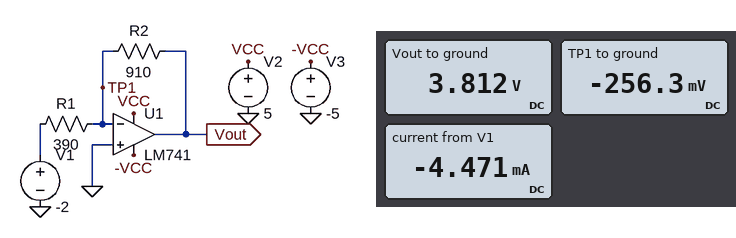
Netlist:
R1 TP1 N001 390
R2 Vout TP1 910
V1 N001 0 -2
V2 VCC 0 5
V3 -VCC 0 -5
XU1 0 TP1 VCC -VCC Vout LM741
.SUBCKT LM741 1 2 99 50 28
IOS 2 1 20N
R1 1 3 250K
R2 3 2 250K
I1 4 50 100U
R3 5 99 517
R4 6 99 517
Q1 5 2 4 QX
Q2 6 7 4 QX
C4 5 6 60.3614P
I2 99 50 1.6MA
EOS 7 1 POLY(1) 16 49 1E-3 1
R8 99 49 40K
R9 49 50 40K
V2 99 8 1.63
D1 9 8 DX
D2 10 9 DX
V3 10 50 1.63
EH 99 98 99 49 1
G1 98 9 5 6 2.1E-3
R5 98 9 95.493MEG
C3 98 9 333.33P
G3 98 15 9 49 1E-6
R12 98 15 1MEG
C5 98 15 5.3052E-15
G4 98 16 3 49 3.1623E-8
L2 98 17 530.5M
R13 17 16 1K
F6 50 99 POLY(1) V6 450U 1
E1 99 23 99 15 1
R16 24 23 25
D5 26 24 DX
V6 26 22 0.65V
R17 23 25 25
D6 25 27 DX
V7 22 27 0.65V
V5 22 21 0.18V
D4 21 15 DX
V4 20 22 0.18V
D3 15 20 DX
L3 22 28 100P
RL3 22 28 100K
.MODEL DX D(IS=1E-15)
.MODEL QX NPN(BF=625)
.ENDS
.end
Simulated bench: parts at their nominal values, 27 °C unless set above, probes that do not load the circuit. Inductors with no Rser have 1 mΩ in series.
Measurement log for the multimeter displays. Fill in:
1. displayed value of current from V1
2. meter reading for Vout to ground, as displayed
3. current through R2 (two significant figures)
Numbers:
-4.471 mA
3.812 V
4.5 mA
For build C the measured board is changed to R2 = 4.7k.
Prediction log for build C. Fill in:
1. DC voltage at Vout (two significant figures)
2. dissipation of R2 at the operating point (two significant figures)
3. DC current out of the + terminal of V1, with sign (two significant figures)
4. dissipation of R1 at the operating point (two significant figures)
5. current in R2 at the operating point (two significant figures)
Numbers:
3.9 V
6.4 mW
-1.2 mA
530 µW
1.2 mA
